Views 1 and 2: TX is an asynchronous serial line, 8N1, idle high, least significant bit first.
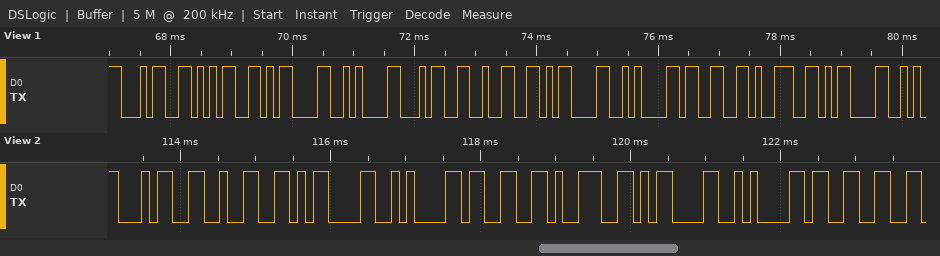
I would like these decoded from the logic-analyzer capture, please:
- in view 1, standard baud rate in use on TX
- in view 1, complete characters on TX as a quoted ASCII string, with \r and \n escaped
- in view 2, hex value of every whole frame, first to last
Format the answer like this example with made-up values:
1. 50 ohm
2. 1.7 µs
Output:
1. 9600 baud
2. "45\r\n42\r\n39\r"
3. 34 32 0D 0A 33 39 0D 0A 33
